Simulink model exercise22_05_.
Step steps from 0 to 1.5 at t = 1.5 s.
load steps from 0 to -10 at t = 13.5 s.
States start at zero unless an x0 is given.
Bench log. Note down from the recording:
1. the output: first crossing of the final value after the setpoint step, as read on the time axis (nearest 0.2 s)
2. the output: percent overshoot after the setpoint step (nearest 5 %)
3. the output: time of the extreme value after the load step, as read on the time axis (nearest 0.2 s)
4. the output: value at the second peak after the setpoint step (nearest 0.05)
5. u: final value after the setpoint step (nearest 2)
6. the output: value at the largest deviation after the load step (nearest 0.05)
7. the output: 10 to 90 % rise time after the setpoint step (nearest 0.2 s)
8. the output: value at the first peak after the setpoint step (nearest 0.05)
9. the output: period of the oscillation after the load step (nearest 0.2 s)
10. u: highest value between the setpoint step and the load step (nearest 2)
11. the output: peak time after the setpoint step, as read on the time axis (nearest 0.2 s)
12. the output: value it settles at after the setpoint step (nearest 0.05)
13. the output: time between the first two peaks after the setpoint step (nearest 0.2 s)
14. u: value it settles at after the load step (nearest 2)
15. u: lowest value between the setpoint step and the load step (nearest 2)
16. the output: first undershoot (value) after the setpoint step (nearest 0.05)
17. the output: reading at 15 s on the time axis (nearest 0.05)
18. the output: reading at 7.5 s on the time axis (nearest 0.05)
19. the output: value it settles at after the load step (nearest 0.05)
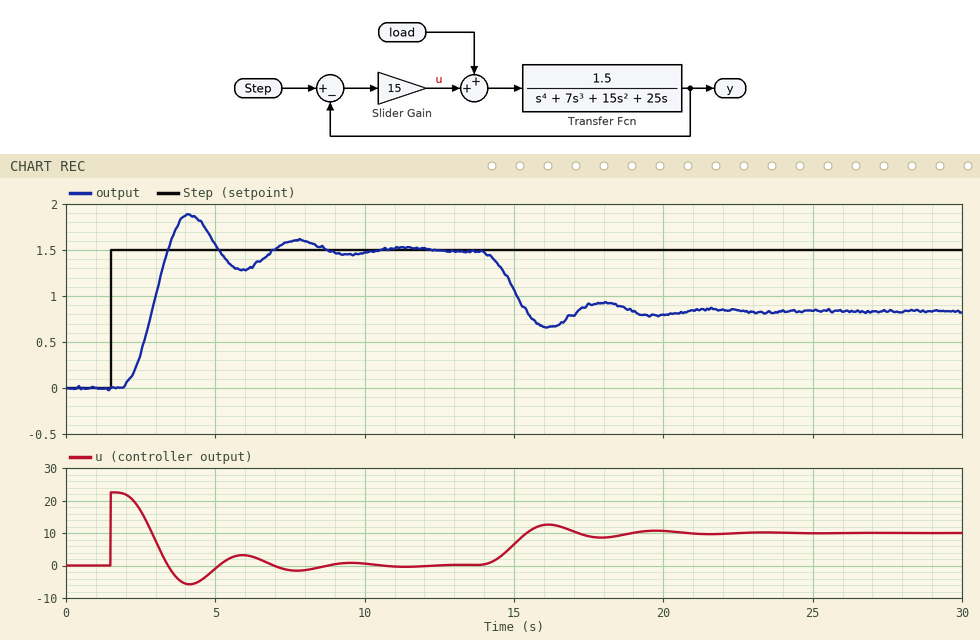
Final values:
3.4 s
25 %
16.2 s
1.60
0
0.65
1.0 s
1.90
3.6 s
22
4.2 s
1.50
3.6 s
10
-6
1.30
1.05
1.60
0.85
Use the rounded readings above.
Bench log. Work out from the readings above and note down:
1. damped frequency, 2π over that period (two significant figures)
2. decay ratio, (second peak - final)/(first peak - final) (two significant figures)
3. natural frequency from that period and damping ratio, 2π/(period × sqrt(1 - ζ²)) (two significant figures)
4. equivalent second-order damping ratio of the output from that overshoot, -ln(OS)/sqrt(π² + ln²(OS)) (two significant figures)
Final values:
1.7 rad/s
0.25
1.9 rad/s
0.40
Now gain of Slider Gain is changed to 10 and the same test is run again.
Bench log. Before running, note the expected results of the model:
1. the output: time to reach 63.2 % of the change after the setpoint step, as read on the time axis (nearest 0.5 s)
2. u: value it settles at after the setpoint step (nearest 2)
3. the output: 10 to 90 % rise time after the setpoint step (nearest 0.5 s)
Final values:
3.5 s
0
1.5 s
